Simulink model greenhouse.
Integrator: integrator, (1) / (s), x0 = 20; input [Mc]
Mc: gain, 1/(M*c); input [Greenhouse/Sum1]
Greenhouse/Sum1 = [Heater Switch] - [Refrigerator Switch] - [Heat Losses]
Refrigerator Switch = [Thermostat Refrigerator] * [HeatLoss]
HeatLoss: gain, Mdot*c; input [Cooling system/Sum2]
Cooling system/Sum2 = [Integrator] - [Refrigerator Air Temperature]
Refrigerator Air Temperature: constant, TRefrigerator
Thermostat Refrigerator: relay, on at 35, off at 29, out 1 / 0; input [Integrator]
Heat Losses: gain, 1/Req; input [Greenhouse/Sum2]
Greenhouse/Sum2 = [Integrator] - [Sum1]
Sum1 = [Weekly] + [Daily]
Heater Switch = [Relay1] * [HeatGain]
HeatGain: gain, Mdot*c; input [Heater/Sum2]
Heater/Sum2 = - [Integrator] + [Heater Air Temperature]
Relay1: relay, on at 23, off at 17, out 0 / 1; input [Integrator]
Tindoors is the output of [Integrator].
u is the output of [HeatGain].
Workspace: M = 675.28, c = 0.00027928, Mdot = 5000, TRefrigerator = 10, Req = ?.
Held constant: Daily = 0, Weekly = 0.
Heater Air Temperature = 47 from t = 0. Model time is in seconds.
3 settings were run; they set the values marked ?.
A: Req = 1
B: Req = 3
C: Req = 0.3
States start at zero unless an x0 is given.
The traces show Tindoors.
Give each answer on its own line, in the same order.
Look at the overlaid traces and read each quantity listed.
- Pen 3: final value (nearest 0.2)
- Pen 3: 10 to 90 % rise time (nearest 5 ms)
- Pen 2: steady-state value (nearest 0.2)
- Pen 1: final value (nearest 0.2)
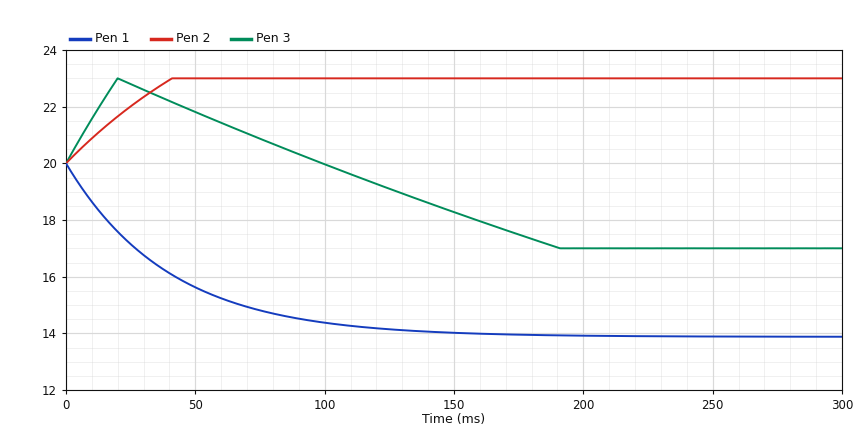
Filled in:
17.0
75 ms
23.0
13.8
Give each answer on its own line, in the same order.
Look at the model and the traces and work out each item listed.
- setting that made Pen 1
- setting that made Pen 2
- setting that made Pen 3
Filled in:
C
A
B
